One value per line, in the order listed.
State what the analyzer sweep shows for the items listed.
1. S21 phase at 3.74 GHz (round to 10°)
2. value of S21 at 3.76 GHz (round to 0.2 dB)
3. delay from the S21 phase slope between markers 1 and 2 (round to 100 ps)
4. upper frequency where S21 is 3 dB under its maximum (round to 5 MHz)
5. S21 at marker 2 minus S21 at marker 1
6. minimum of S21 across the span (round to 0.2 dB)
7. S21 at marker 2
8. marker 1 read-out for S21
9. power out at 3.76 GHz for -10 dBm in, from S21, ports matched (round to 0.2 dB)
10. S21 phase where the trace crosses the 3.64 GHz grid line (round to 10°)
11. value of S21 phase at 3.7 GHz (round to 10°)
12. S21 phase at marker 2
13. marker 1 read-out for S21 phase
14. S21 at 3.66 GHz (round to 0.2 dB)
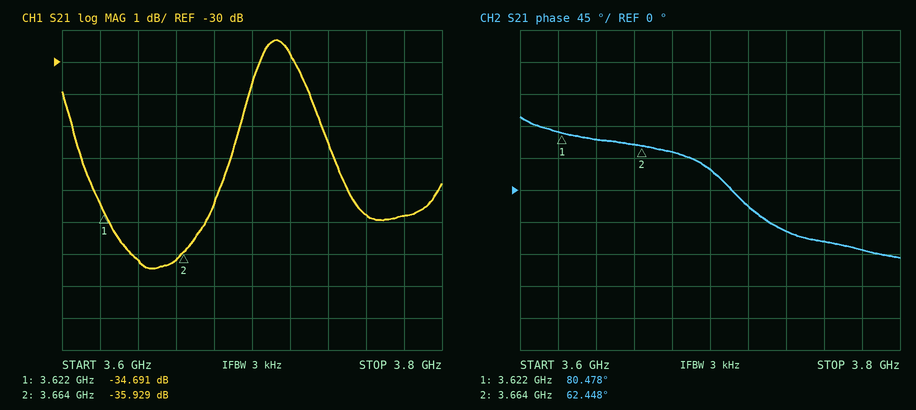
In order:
-60°
-34.8 dB
1.2 ns
3.740 GHz
-1.238 dB
-36.4 dB
-35.929 dB
-34.691 dB
-44.8 dBm
70°
30°
62.448°
80.478°
-36.2 dB
